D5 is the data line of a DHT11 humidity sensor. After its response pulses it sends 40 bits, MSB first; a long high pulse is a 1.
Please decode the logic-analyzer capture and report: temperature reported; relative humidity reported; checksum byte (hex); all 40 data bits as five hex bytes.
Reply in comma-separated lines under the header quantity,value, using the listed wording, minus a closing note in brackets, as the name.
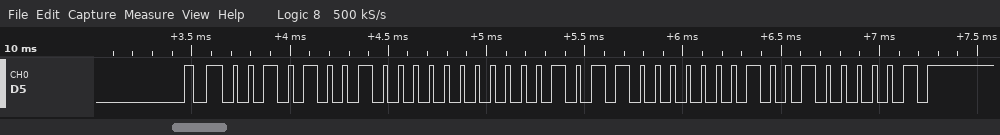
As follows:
quantity,value
temperature reported,22.2 °C
relative humidity reported,41 %
checksum byte,0x41
all 40 data bits as five hex bytes,29 00 16 02 41
